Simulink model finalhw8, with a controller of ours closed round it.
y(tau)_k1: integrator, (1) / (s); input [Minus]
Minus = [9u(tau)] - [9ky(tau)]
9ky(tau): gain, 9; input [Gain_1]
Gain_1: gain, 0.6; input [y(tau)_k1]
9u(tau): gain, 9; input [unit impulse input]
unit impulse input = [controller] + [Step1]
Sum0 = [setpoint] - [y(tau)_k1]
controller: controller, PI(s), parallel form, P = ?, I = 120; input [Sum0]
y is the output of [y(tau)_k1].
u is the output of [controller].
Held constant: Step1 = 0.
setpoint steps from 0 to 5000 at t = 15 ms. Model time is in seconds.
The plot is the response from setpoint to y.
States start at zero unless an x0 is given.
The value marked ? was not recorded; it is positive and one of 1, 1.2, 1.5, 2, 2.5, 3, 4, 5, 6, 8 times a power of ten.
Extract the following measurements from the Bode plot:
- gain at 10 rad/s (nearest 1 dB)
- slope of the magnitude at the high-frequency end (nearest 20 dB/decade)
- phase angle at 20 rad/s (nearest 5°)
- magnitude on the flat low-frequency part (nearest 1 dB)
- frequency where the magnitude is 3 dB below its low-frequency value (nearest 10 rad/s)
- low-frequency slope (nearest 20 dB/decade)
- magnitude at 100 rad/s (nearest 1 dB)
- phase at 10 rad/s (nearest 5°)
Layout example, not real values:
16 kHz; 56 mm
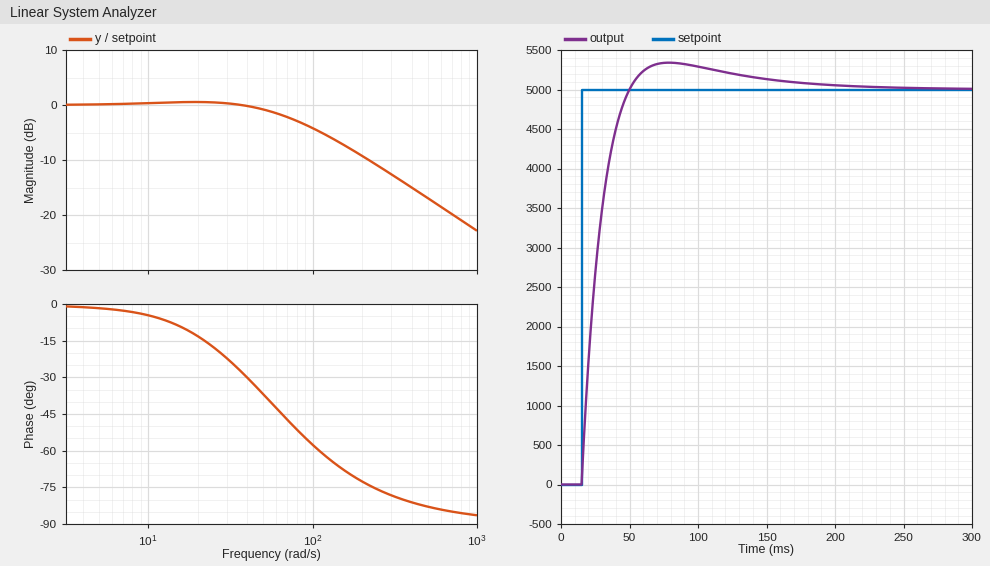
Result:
0 dB; -20 dB/decade; -15°; 0 dB; 80 rad/s; 0 dB/decade; -4 dB; -5°
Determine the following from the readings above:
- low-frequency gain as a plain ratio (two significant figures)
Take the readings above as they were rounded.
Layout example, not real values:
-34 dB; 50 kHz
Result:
1.0
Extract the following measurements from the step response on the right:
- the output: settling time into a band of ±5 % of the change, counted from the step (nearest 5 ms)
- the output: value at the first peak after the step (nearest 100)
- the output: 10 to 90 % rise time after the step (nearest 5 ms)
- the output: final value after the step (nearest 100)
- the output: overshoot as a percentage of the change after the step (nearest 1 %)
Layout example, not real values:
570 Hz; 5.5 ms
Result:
95 ms; 5300; 25 ms; 5000; 7 %
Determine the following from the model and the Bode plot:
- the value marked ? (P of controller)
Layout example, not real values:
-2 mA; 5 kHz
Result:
8
